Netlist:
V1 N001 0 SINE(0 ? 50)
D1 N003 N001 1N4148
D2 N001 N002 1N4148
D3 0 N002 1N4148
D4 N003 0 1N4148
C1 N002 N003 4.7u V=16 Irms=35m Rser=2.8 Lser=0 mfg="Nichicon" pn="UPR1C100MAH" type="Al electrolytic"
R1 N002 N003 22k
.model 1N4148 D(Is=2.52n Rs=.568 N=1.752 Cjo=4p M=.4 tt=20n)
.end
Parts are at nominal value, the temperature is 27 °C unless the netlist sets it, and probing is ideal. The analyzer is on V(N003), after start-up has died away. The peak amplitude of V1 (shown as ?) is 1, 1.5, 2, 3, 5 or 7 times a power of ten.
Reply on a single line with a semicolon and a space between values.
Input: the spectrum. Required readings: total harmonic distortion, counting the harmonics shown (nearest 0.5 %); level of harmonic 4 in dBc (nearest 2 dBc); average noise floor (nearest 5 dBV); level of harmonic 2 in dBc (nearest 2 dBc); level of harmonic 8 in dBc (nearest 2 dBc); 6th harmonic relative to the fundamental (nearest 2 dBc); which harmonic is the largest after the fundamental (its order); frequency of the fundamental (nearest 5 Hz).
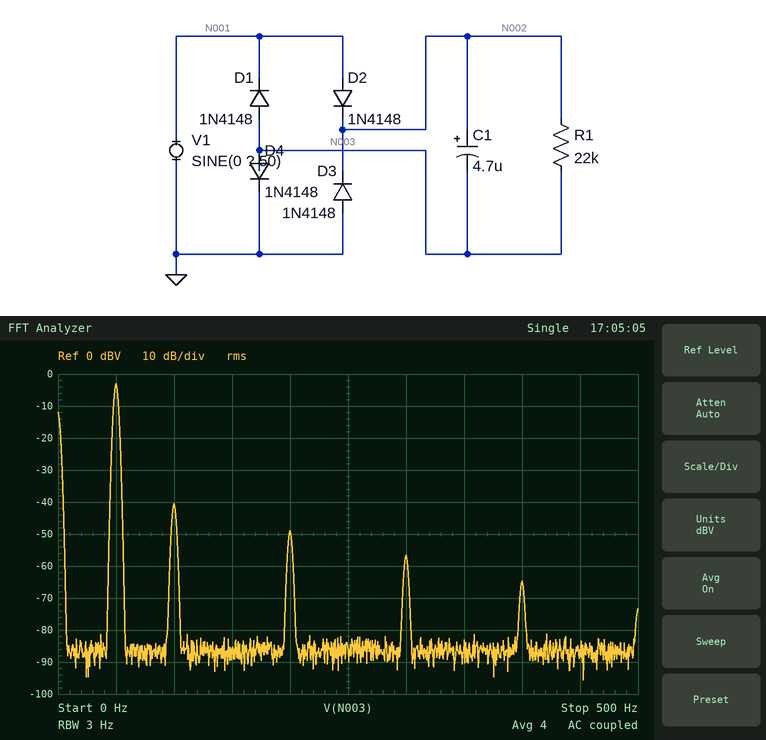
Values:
1.5 %; -46 dBc; -85 dBV; -38 dBc; -62 dBc; -54 dBc; 2; 50 Hz
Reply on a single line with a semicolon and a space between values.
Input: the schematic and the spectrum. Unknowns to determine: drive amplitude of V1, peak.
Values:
2 V
